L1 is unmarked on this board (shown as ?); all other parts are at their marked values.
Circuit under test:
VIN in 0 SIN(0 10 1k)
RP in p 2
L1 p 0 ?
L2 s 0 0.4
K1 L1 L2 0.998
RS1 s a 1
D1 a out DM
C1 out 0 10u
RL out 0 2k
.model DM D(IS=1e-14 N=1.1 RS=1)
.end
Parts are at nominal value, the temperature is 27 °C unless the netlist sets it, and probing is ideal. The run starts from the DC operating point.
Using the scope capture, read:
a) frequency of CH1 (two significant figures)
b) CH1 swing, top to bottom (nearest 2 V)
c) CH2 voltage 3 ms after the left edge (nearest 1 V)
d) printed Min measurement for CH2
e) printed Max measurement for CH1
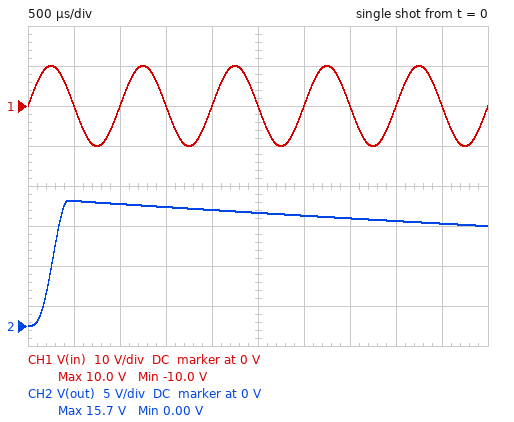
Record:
1.0 kHz
20 V
14 V
0.00 V
10.0 V
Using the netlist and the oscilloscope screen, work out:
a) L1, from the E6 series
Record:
220 mH
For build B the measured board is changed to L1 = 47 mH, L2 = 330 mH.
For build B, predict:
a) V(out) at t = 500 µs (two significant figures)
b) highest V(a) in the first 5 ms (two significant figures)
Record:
21 V
24 V
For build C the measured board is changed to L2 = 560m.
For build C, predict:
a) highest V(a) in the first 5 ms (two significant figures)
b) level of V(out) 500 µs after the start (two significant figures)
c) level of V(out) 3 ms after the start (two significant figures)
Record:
18 V
17 V
15 V
